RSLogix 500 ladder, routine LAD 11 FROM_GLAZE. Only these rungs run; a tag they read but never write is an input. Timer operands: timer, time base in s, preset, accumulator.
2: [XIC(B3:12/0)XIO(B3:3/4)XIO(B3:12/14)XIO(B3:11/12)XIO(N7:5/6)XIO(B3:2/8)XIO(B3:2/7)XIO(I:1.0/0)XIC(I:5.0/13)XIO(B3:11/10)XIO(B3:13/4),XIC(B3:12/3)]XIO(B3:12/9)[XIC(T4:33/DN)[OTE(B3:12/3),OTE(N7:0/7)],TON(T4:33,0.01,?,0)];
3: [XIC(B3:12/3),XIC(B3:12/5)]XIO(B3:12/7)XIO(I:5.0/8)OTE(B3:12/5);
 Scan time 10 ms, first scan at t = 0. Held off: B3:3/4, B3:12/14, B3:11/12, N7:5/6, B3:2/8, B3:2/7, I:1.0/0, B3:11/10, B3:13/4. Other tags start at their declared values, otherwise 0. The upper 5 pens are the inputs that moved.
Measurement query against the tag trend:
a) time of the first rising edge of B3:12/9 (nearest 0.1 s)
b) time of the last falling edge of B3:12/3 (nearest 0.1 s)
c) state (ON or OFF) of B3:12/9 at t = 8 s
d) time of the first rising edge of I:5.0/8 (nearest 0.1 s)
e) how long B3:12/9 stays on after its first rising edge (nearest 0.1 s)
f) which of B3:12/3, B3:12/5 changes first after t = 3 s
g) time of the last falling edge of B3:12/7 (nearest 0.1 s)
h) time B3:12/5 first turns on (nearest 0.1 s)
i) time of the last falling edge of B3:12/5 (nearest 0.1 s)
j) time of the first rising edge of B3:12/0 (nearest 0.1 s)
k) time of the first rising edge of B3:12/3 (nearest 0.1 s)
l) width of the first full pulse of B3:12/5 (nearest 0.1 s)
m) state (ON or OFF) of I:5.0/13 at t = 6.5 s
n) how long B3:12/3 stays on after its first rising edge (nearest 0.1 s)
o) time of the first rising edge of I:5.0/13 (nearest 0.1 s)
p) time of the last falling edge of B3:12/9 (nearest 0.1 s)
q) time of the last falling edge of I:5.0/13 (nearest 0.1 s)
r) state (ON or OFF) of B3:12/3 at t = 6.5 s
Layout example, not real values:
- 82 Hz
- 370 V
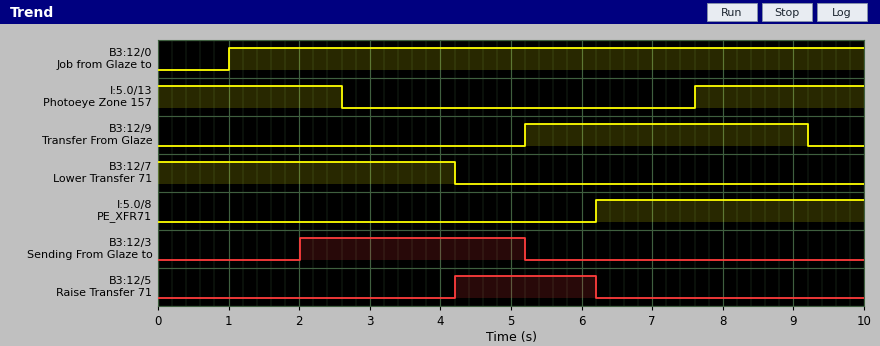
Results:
- 5.2 s
- 5.2 s
- ON
- 6.2 s
- 4.0 s
- B3:12/5
- 4.2 s
- 4.2 s
- 6.2 s
- 1.0 s
- 2.0 s
- 2.0 s
- OFF
- 3.2 s
- 7.6 s
- 9.2 s
- 2.6 s
- OFF
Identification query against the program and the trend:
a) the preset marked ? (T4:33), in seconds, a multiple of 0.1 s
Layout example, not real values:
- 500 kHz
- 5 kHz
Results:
- 1.0 s
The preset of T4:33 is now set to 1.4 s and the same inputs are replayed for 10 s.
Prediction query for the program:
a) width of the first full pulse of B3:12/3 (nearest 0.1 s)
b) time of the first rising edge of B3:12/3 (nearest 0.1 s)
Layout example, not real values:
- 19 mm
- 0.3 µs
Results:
- 2.8 s
- 2.4 s
